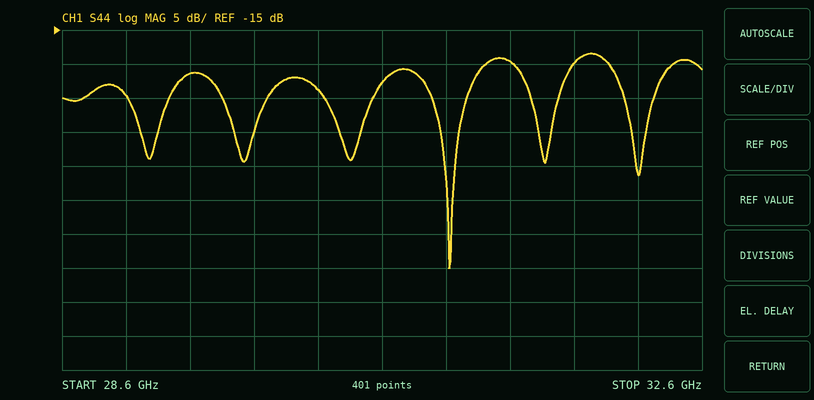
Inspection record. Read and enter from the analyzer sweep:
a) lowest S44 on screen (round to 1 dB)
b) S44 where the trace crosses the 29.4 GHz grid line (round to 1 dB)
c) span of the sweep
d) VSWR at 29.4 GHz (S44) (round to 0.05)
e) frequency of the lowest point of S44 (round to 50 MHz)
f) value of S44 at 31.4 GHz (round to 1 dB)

-50 dB
-21 dB
4 GHz
1.20
31.00 GHz
-20 dB
